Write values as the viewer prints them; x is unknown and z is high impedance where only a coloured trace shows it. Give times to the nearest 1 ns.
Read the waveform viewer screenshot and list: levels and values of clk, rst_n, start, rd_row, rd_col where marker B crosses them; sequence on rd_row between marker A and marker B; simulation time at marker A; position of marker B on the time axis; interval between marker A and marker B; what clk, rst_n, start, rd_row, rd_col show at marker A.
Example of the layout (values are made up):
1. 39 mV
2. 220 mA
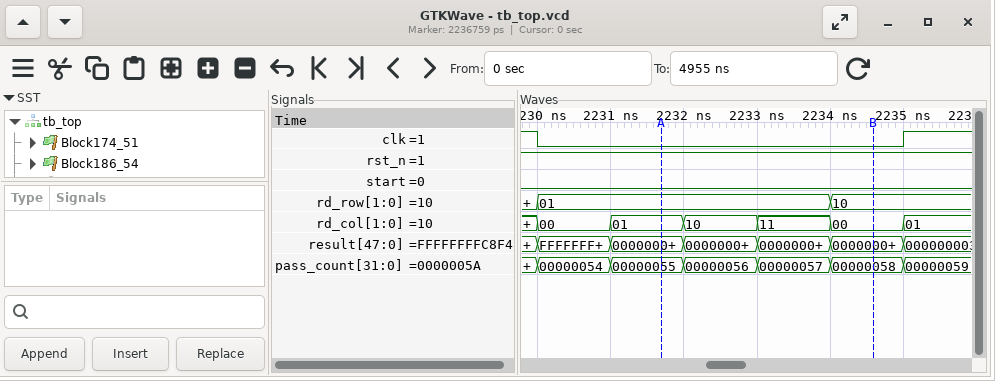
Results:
1. clk=0, rst_n=1, start=0, rd_row=10, rd_col=00
2. 01, 10
3. 2232 ns
4. 2235 ns
5. 3 ns
6. clk=0, rst_n=1, start=0, rd_row=01, rd_col=01
